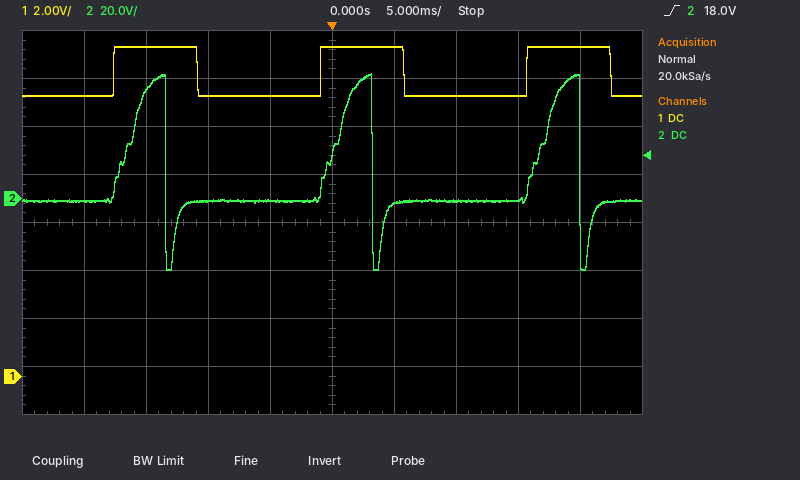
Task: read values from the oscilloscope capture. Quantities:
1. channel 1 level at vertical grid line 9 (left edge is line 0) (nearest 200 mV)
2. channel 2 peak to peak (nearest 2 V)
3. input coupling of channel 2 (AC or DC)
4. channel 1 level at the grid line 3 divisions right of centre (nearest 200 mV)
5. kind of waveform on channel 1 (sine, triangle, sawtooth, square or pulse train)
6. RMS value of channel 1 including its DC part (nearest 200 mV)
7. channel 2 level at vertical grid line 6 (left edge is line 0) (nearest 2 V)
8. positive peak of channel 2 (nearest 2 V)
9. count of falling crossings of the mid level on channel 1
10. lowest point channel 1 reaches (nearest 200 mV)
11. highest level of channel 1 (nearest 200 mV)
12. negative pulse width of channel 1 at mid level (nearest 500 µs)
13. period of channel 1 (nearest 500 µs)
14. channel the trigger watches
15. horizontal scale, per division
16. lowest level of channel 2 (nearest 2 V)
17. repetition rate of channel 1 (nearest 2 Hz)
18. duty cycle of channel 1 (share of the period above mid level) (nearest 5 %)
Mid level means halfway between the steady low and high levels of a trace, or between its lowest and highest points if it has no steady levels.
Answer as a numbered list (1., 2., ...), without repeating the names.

1. 13.8 V
2. 82 V
3. DC
4. 11.6 V
5. pulse train
6. 12.6 V
7. -2 V
8. 52 V
9. 3
10. 11.6 V
11. 13.8 V
12. 10.0 ms
13. 16.5 ms
14. channel 2
15. 5 ms
16. -30 V
17. 60 Hz
18. 40 %
